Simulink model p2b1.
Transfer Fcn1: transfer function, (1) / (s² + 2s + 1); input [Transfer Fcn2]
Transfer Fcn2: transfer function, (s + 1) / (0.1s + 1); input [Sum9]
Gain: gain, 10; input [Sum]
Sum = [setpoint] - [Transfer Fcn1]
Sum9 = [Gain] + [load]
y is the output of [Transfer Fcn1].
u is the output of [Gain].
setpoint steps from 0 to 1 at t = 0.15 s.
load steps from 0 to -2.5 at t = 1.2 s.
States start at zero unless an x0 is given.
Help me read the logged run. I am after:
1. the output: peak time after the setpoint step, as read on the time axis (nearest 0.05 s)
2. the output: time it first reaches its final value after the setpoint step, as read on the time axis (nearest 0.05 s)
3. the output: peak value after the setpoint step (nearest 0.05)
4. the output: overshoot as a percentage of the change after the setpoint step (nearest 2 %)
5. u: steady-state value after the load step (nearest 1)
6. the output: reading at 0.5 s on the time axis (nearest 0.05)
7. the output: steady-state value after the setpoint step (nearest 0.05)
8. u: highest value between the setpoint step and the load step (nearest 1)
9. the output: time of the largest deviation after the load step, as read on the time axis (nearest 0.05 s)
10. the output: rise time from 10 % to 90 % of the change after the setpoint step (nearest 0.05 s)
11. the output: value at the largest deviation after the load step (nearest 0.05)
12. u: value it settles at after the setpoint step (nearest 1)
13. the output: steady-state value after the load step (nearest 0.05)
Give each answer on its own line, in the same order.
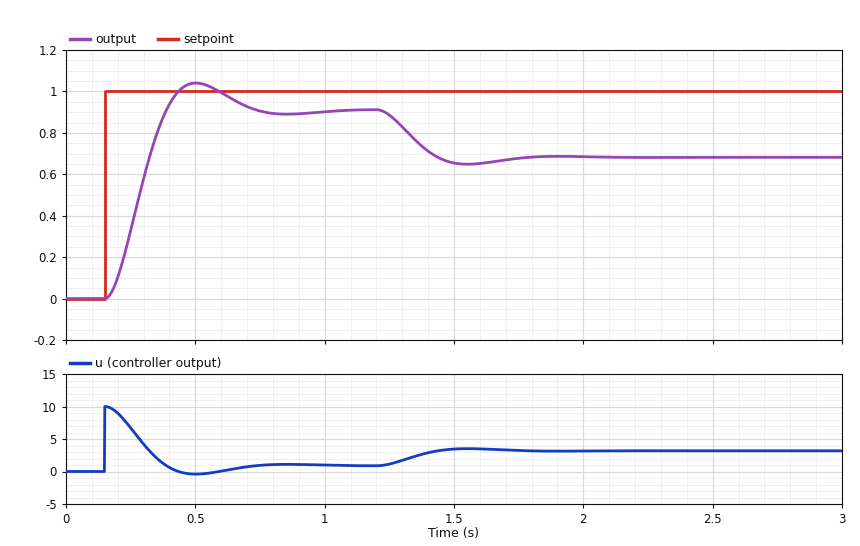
0.50 s
0.40 s
1.05
14 %
3
1.05
0.90
10
1.55 s
0.15 s
0.65
1
0.70
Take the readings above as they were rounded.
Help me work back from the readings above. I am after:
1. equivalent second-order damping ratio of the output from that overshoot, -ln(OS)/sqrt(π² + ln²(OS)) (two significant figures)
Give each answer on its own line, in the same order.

0.53
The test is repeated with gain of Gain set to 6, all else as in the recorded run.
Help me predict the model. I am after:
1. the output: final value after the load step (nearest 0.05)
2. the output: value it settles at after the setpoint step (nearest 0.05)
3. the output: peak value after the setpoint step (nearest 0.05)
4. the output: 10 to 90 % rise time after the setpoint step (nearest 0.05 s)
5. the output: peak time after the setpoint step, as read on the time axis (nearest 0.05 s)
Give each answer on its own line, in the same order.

0.50
0.85
0.90
0.25 s
0.65 s
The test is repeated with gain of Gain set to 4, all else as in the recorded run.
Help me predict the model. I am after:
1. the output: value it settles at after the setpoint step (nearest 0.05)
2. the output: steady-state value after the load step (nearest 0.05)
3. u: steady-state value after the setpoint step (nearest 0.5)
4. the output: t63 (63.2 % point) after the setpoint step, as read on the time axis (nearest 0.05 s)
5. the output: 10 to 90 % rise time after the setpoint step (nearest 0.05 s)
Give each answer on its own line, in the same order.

0.80
0.30
1.0
0.40 s
0.35 s
